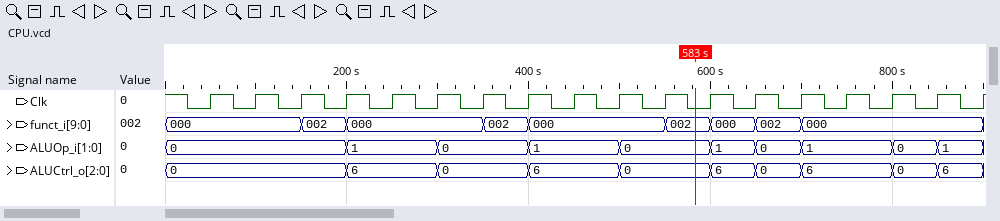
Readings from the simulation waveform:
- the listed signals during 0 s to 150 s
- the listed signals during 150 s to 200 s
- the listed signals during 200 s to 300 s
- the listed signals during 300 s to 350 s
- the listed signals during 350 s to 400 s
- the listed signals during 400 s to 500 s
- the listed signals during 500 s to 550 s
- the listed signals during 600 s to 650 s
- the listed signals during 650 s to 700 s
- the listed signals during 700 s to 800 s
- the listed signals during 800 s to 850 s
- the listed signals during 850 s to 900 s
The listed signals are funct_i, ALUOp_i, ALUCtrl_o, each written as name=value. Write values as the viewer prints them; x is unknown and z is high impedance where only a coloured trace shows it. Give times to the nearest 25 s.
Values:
funct_i=000, ALUOp_i=0, ALUCtrl_o=0
funct_i=002, ALUOp_i=0, ALUCtrl_o=0
funct_i=000, ALUOp_i=1, ALUCtrl_o=6
funct_i=000, ALUOp_i=0, ALUCtrl_o=0
funct_i=002, ALUOp_i=0, ALUCtrl_o=0
funct_i=000, ALUOp_i=1, ALUCtrl_o=6
funct_i=000, ALUOp_i=0, ALUCtrl_o=0
funct_i=000, ALUOp_i=1, ALUCtrl_o=6
funct_i=002, ALUOp_i=0, ALUCtrl_o=0
funct_i=000, ALUOp_i=1, ALUCtrl_o=6
funct_i=000, ALUOp_i=0, ALUCtrl_o=0
funct_i=000, ALUOp_i=1, ALUCtrl_o=6
